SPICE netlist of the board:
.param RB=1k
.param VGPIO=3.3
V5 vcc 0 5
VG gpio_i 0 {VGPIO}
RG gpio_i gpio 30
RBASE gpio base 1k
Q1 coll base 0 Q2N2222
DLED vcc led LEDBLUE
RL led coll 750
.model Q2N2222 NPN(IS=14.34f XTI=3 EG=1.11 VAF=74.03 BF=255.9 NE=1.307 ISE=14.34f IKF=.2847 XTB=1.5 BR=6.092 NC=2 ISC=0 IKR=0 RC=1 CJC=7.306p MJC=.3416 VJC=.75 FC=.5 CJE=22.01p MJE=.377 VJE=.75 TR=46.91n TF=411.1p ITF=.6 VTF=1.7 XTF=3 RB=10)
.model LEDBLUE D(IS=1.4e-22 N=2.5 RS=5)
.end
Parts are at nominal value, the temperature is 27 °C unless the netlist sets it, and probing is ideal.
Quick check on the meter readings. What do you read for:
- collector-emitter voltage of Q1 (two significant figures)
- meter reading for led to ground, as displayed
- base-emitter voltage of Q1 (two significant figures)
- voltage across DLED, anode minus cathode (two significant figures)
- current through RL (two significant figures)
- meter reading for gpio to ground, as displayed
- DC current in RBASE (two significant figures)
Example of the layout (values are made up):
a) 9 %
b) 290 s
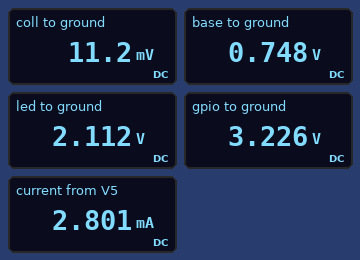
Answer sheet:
a) 11 mV
b) 2.112 V
c) 750 mV
d) 2.9 V
e) 2.8 mA
f) 3.226 V
g) 2.5 mA
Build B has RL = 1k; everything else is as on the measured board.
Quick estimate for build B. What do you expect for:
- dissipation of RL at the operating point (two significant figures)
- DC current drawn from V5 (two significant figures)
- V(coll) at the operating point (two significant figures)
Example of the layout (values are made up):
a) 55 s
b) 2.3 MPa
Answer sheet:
a) 4.5 mW
b) 2.1 mA
c) 9.6 mV
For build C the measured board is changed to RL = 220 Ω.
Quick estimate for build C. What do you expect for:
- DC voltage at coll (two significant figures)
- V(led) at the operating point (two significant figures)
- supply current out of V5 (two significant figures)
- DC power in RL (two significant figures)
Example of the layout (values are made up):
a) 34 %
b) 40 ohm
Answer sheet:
a) 25 mV
b) 2.0 V
c) 9.0 mA
d) 18 mW
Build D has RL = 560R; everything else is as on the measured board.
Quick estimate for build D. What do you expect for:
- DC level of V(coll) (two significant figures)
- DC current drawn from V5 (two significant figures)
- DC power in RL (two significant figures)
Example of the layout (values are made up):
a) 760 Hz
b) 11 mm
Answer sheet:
a) 13 mV
b) 3.7 mA
c) 7.7 mW
